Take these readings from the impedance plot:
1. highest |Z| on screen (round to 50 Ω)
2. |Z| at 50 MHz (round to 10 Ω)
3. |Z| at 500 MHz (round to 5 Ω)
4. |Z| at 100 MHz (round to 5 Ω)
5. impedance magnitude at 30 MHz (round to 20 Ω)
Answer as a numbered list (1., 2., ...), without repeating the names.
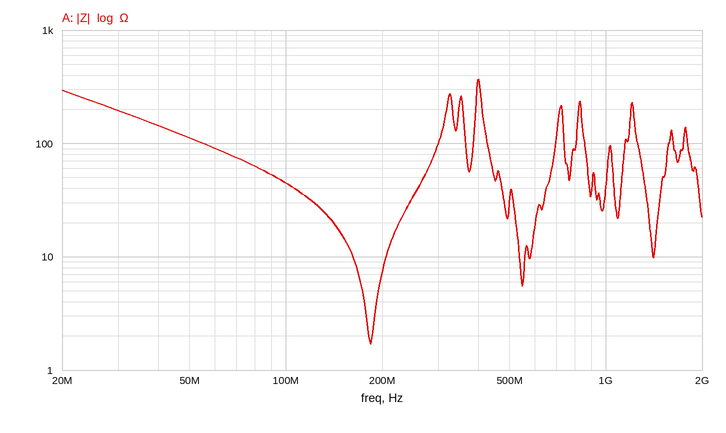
1. 350 Ω
2. 110 Ω
3. 30 Ω
4. 45 Ω
5. 200 Ω
